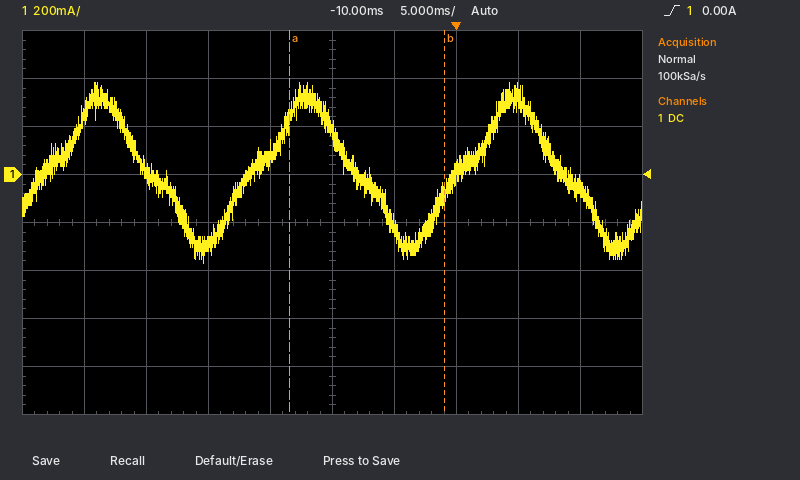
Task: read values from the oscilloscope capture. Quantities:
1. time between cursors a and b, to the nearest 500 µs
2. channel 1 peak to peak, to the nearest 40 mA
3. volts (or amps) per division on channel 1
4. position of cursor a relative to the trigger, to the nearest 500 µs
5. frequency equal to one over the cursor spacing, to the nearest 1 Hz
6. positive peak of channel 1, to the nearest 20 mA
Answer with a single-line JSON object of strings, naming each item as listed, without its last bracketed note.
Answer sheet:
{"time between cursors a and b, to the nearest 500 µs": "12.5 ms", "channel 1 peak to peak, to the nearest 40 mA": "760 mA", "volts (or amps) per division on channel 1": "200 mA", "position of cursor a relative to the trigger, to the nearest 500 µs": "-13.5 ms", "frequency equal to one over the cursor spacing, to the nearest 1 Hz": "80 Hz", "positive peak of channel 1, to the nearest 20 mA": "380 mA"}
